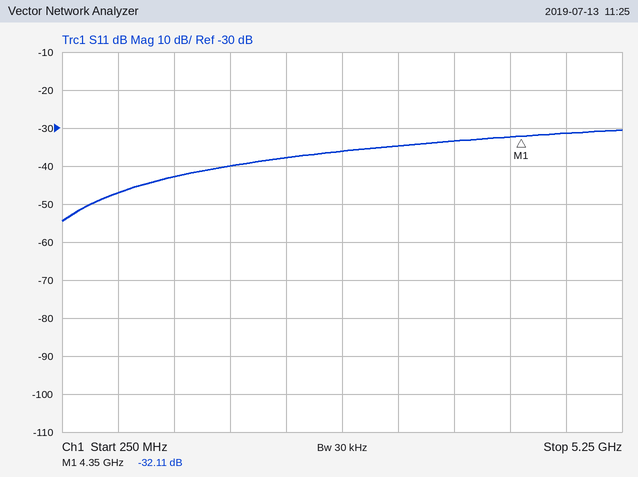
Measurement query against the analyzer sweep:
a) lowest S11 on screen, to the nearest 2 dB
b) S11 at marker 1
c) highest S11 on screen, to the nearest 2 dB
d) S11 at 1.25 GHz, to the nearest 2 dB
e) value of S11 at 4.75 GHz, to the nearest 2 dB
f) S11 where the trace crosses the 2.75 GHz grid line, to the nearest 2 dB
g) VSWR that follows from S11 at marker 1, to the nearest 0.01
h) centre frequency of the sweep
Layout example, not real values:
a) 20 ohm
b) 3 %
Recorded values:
a) -54 dB
b) -32.11 dB
c) -30 dB
d) -42 dB
e) -32 dB
f) -36 dB
g) 1.05
h) 2.75 GHz
